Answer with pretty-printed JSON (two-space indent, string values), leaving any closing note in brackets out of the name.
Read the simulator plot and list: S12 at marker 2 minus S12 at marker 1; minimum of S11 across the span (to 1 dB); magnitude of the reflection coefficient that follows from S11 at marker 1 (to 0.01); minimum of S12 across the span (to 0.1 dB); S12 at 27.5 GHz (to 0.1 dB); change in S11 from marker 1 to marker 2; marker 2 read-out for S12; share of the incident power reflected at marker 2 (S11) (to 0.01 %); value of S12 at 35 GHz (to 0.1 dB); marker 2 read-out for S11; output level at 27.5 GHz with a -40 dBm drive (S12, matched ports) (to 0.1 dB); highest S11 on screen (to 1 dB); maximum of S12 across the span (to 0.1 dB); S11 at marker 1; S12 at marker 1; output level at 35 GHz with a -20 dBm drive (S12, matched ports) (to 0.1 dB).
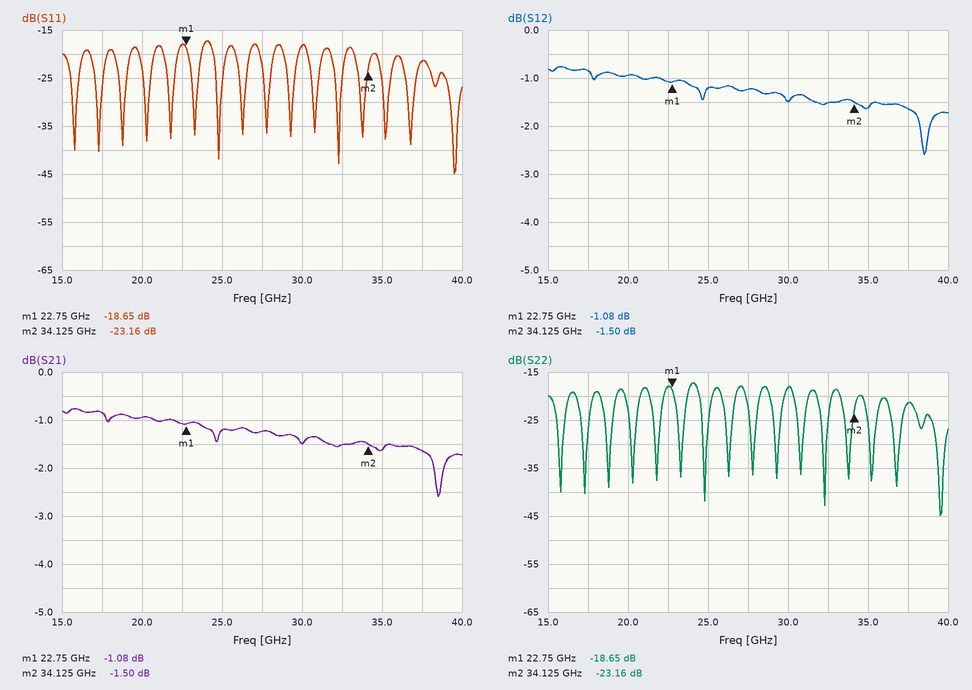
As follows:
{
  "S12 at marker 2 minus S12 at marker 1": "-0.42 dB",
  "minimum of S11 across the span": "-45 dB",
  "magnitude of the reflection coefficient that follows from S11 at marker 1": "0.12",
  "minimum of S12 across the span": "-2.6 dB",
  "S12 at 27.5 GHz": "-1.2 dB",
  "change in S11 from marker 1 to marker 2": "-4.51 dB",
  "marker 2 read-out for S12": "-1.50 dB",
  "share of the incident power reflected at marker 2 (S11)": "0.48 %",
  "value of S12 at 35 GHz": "-1.6 dB",
  "marker 2 read-out for S11": "-23.16 dB",
  "output level at 27.5 GHz with a -40 dBm drive (S12, matched ports)": "-41.2 dBm",
  "highest S11 on screen": "-17 dB",
  "maximum of S12 across the span": "-0.8 dB",
  "S11 at marker 1": "-18.65 dB",
  "S12 at marker 1": "-1.08 dB",
  "output level at 35 GHz with a -20 dBm drive (S12, matched ports)": "-21.6 dBm"
}
